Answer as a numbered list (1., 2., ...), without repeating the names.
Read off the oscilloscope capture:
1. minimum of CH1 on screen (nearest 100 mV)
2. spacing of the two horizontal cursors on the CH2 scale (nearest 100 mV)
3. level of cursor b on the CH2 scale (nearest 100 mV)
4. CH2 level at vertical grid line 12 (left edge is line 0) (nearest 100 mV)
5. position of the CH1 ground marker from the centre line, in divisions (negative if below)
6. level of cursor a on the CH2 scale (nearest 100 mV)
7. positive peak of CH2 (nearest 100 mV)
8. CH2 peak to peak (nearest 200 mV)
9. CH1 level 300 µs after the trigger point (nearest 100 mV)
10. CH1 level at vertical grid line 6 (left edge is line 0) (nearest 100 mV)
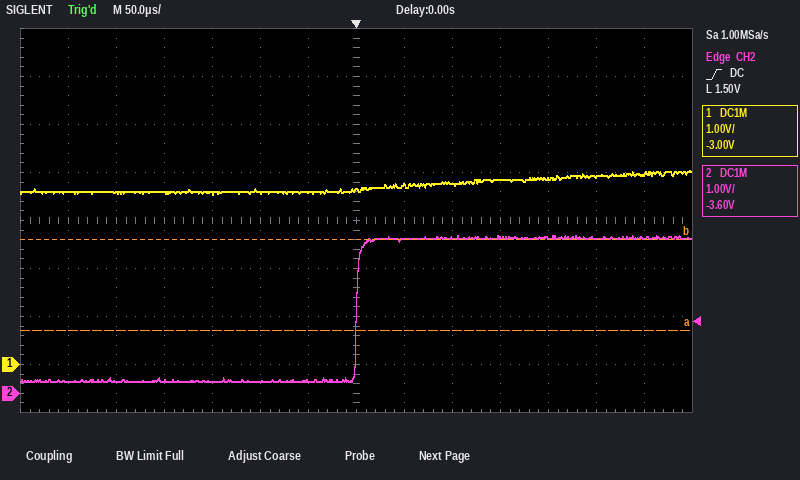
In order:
1. 3.5 V
2. 1.9 V
3. 3.2 V
4. 3.2 V
5. -3.0 div
6. 1.3 V
7. 3.3 V
8. 3.0 V
9. 4.0 V
10. 3.6 V
